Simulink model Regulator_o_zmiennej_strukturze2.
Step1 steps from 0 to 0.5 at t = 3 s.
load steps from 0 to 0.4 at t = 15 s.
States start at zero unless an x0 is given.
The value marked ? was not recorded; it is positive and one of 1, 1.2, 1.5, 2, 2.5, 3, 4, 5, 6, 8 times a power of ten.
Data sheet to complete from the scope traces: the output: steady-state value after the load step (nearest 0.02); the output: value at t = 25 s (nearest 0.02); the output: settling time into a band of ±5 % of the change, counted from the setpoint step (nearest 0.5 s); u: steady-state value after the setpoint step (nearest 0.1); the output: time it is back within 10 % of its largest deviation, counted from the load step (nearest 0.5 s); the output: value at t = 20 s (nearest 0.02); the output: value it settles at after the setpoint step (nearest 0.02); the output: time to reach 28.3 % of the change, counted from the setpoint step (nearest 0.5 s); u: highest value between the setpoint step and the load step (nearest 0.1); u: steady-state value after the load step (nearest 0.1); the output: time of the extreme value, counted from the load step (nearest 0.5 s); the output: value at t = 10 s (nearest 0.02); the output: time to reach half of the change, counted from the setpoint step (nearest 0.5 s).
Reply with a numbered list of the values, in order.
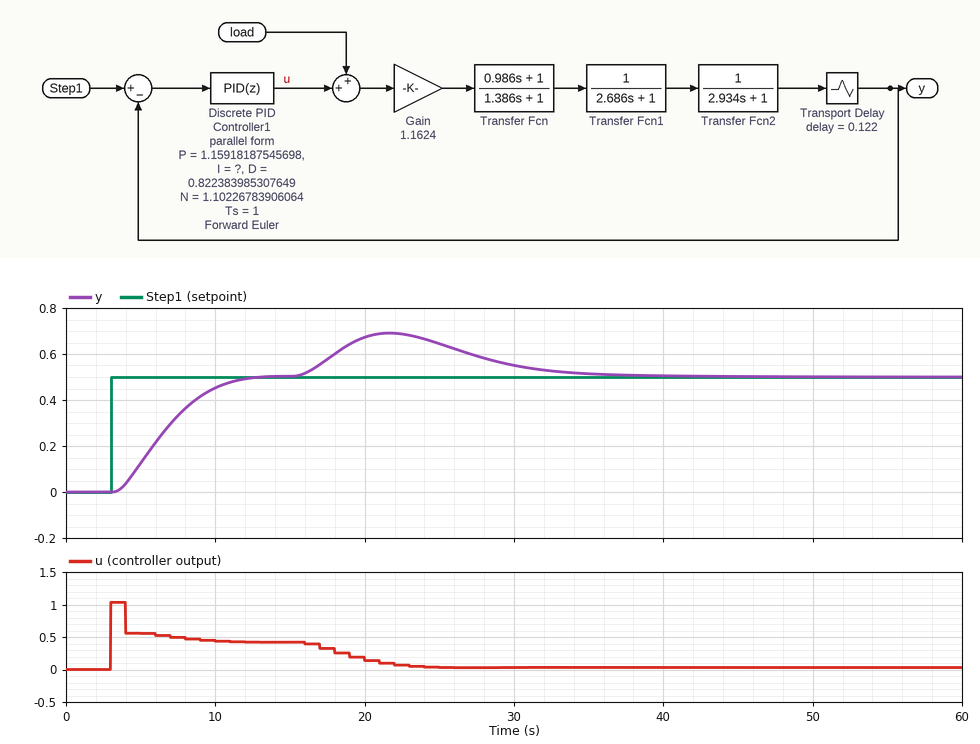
1. 0.50
2. 0.64
3. 8.0 s
4. 0.4
5. 19.0 s
6. 0.68
7. 0.50
8. 2.0 s
9. 1.0
10. 0.0
11. 6.5 s
12. 0.46
13. 3.5 s
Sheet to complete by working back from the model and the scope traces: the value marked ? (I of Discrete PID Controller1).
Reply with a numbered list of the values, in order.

1. 0.2
